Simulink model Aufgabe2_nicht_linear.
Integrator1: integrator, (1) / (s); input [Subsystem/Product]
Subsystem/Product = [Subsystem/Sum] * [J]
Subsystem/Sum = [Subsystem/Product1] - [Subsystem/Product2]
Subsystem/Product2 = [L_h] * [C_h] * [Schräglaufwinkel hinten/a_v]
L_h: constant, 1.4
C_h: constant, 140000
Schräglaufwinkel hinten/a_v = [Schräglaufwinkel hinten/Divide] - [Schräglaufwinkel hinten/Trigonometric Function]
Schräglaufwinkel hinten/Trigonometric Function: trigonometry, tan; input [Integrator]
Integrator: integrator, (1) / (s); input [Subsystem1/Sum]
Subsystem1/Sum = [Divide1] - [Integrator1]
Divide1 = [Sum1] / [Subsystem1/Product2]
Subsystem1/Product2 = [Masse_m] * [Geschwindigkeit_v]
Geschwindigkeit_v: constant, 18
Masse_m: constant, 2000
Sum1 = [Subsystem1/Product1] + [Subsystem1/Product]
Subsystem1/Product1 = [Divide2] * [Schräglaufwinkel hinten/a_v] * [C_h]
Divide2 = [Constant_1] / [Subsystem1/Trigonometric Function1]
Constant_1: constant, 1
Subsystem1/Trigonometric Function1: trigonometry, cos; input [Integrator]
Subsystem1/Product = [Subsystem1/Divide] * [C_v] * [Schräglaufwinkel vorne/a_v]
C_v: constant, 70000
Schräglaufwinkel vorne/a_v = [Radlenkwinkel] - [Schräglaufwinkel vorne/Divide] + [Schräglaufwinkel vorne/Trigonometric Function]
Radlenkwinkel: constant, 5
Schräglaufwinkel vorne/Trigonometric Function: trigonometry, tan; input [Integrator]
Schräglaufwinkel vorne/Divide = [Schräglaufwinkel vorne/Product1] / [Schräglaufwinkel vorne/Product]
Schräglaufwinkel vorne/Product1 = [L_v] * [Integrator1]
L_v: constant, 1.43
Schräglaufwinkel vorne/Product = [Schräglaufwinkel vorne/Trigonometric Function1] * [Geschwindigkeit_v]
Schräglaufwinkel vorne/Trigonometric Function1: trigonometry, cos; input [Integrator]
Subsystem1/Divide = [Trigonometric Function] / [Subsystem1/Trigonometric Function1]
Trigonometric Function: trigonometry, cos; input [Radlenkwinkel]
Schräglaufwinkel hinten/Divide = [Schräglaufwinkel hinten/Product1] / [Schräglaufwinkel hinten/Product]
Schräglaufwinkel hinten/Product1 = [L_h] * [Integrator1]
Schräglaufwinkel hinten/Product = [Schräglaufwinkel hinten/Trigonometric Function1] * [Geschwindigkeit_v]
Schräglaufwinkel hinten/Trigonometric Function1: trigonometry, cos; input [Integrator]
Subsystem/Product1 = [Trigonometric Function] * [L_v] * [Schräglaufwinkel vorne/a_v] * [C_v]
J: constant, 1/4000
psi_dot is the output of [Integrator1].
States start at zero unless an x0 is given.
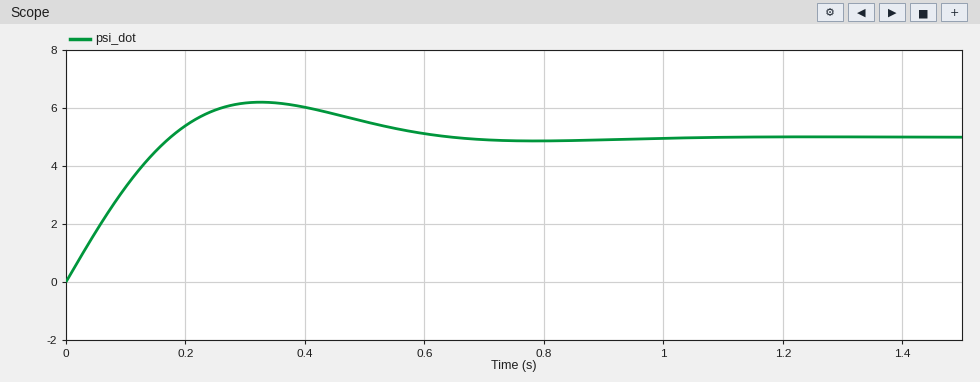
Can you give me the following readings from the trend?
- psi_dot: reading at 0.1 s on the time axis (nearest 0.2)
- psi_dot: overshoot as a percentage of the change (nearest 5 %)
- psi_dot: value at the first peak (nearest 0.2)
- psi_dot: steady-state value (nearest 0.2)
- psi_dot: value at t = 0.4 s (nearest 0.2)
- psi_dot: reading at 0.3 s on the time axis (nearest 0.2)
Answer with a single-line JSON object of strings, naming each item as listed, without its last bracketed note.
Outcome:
{"psi_dot: reading at 0.1 s on the time axis": "3.2", "psi_dot: overshoot as a percentage of the change": "25 %", "psi_dot: value at the first peak": "6.2", "psi_dot: steady-state value": "5.0", "psi_dot: value at t = 0.4 s": "6.0", "psi_dot: reading at 0.3 s on the time axis": "6.2"}
